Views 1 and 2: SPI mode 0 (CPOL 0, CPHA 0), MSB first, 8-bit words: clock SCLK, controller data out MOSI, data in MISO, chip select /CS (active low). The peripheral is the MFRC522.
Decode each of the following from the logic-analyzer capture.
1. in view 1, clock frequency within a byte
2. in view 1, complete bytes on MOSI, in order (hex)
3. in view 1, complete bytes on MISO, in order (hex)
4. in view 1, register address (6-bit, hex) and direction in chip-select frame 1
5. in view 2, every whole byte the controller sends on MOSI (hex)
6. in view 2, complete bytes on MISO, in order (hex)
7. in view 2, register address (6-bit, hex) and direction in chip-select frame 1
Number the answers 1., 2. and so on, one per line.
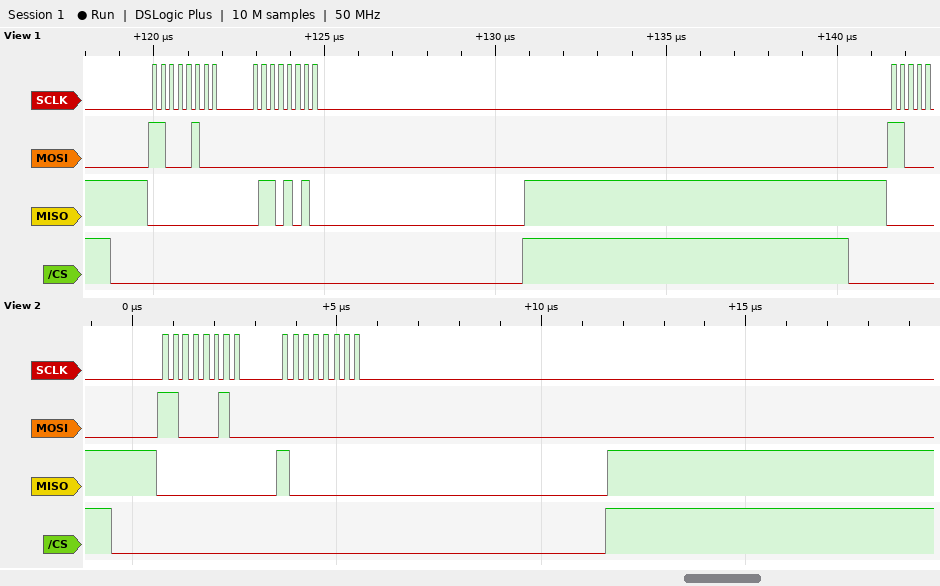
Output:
1. 4 MHz
2. C4 00
3. 00 6A
4. 0x22 read
5. 0xC2 0x00
6. 0x00 0x80
7. 0x21 read
